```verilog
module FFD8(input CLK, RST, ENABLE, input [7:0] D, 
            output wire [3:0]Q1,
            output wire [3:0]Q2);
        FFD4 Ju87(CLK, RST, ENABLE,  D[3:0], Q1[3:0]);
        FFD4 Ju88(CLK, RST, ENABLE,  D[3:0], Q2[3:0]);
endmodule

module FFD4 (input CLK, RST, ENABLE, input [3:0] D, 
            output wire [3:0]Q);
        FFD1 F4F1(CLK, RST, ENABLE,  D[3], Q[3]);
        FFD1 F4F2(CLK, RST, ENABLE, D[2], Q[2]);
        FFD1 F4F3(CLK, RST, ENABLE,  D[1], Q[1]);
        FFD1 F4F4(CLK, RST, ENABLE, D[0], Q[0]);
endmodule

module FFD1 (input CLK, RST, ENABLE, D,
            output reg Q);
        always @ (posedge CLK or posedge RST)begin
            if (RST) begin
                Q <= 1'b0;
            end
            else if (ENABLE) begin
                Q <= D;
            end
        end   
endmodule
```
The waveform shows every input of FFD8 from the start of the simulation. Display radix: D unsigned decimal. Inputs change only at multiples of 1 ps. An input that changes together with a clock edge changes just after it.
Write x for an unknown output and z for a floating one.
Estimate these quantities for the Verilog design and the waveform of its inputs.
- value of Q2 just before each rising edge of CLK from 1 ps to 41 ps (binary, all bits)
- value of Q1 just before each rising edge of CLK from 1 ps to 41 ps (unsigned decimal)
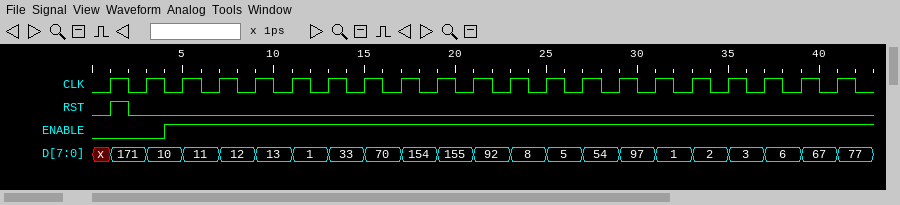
x, 0000, 0000, 1010, 1011, 1100, 1101, 0001, 0001, 0110, 1010, 1011, 1100, 1000, 0101, 0110, 0001, 0001, 0010, 0011, 0110
x, 0, 0, 10, 11, 12, 13, 1, 1, 6, 10, 11, 12, 8, 5, 6, 1, 1, 2, 3, 6
